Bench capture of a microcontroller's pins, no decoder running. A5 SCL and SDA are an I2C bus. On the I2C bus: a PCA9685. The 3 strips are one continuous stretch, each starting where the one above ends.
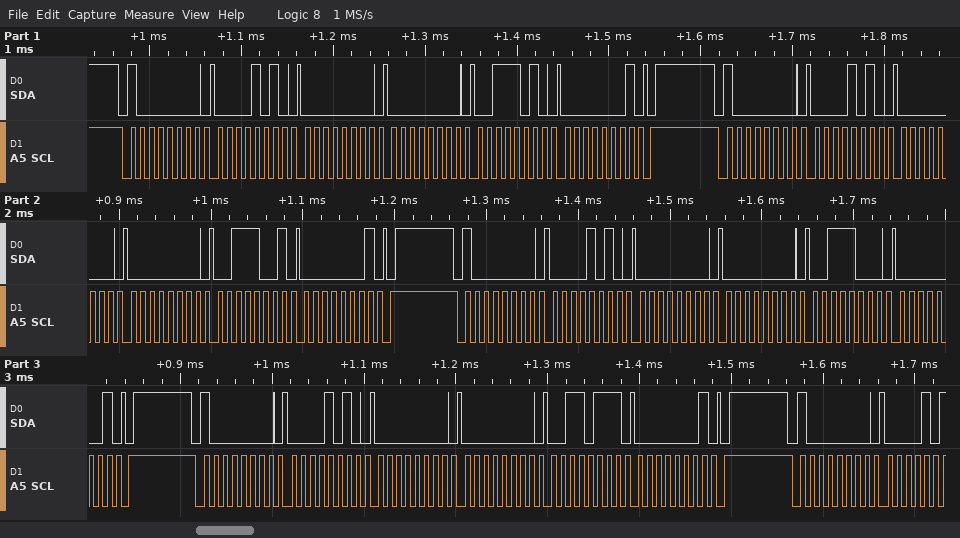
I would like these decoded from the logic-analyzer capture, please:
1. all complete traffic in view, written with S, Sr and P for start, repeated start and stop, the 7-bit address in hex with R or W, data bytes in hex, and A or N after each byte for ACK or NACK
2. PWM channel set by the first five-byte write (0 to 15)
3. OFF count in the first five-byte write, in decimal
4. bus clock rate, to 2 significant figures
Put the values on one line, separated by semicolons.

S 40W A 0A A 00 A 00 A 3A A 01 A P S 40W A 0A A 00 A 00 A 39 A 01 A P S 40W A 0A A 00 A 00 A 38 A 01 A P S 40W A 0A A 00 A 00 A 37 A 01 A P S 40W A; 1; 314; 100 kHz
